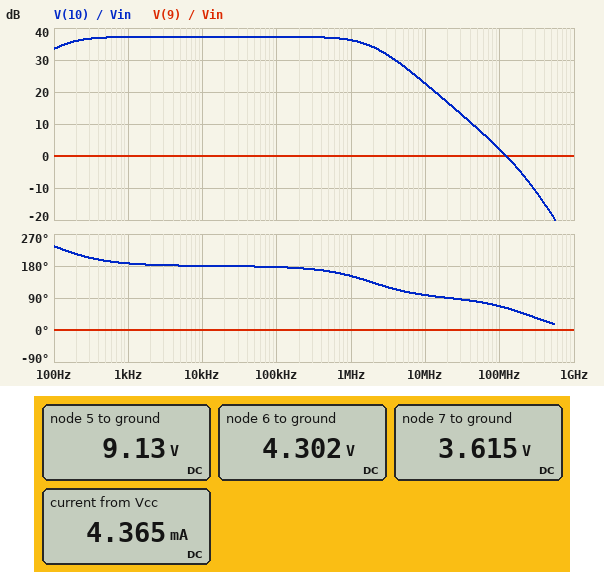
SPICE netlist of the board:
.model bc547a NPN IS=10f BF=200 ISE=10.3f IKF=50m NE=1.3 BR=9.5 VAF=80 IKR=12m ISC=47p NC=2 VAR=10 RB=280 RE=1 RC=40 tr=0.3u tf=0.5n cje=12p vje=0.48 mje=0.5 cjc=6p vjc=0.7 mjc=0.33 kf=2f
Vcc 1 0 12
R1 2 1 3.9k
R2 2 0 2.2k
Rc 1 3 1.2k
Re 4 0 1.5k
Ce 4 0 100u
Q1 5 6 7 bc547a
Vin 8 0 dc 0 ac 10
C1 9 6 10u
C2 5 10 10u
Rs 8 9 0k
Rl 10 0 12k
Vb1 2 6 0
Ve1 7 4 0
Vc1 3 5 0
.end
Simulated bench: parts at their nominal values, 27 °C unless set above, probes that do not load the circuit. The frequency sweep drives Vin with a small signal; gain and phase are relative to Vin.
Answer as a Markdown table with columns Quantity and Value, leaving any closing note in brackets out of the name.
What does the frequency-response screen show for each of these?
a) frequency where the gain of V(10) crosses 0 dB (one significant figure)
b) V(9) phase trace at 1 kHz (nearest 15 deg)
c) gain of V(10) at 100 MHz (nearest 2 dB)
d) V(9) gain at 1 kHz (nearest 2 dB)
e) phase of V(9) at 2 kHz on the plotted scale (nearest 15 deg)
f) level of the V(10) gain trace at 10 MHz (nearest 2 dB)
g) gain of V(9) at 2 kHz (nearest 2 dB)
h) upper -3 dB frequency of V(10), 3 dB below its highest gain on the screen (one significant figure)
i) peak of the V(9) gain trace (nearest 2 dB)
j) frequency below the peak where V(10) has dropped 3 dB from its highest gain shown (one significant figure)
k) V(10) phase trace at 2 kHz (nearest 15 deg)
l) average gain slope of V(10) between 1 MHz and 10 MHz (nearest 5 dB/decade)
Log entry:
| Quantity | Value |
|---|---|
| frequency where the gain of V(10) crosses 0 dB | 100 MHz |
| V(9) phase trace at 1 kHz | 0 deg |
| gain of V(10) at 100 MHz | 2 dB |
| V(9) gain at 1 kHz | 0 dB |
| phase of V(9) at 2 kHz on the plotted scale | 0 deg |
| level of the V(10) gain trace at 10 MHz | 22 dB |
| gain of V(9) at 2 kHz | 0 dB |
| upper -3 dB frequency of V(10), 3 dB below its highest gain on the screen | 2 MHz |
| peak of the V(9) gain trace | 0 dB |
| frequency below the peak where V(10) has dropped 3 dB from its highest gain shown | 100 Hz |
| V(10) phase trace at 2 kHz | 180 deg |
| average gain slope of V(10) between 1 MHz and 10 MHz | -15 dB/decade |
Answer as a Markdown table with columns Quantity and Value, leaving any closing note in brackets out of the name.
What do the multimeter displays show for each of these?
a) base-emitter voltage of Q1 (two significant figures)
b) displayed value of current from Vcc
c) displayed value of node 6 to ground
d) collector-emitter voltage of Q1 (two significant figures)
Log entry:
| Quantity | Value |
|---|---|
| base-emitter voltage of Q1 | 690 mV |
| displayed value of current from Vcc | 4.365 mA |
| displayed value of node 6 to ground | 4.302 V |
| collector-emitter voltage of Q1 | 5.5 V |
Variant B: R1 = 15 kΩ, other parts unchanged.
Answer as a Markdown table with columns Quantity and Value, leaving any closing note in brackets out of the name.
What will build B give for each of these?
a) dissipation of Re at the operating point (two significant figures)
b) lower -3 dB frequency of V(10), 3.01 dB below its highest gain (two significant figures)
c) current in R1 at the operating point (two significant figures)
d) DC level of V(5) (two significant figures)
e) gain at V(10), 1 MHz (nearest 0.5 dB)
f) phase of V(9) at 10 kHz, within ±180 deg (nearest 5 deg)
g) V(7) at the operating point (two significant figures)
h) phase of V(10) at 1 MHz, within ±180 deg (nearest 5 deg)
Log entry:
| Quantity | Value |
|---|---|
| dissipation of Re at the operating point | 520 µW |
| lower -3 dB frequency of V(10), 3.01 dB below its highest gain | 39 Hz |
| current in R1 at the operating point | 700 µA |
| DC level of V(5) | 11 V |
| gain at V(10), 1 MHz | 27.0 dB |
| phase of V(9) at 10 kHz, within ±180 deg | 0 deg |
| V(7) at the operating point | 880 mV |
| phase of V(10) at 1 MHz, within ±180 deg | 170 deg |
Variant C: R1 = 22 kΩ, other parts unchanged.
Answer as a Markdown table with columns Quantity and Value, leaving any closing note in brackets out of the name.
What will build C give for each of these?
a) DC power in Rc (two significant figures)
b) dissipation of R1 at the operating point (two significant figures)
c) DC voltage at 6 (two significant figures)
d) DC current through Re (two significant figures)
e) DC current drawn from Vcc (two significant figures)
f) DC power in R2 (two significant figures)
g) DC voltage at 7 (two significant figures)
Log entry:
| Quantity | Value |
|---|---|
| DC power in Rc | 110 µW |
| dissipation of R1 at the operating point | 5.4 mW |
| DC voltage at 6 | 1.1 V |
| DC current through Re | 310 µA |
| DC current drawn from Vcc | 800 µA |
| DC power in R2 | 540 µW |
| DC voltage at 7 | 460 mV |
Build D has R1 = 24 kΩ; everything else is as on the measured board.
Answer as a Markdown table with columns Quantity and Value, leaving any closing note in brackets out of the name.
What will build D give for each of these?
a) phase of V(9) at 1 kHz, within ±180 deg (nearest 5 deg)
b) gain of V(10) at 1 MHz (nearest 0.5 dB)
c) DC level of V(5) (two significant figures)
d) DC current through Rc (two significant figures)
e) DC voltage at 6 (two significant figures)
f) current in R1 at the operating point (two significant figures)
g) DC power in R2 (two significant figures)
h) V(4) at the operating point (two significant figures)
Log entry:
| Quantity | Value |
|---|---|
| phase of V(9) at 1 kHz, within ±180 deg | 0 deg |
| gain of V(10) at 1 MHz | 20.0 dB |
| DC level of V(5) | 12 V |
| DC current through Rc | 250 µA |
| DC voltage at 6 | 1.0 V |
| current in R1 at the operating point | 460 µA |
| DC power in R2 | 460 µW |
| V(4) at the operating point | 380 mV |
